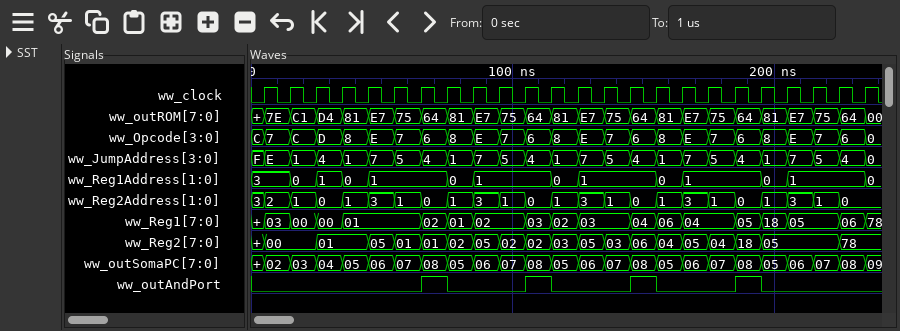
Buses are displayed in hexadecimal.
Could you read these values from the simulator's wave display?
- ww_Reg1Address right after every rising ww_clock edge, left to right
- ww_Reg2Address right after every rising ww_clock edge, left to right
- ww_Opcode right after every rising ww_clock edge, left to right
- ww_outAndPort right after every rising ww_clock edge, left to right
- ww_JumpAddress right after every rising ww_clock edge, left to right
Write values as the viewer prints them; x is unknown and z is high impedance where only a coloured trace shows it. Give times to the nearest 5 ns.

3, 0, 1, 0, 1, 1, 1, 0, 1, 1, 1, 0, 1, 1, 1, 0, 1, 1, 1, 0, 1, 1, 1, 0
2, 1, 0, 1, 3, 1, 0, 1, 3, 1, 0, 1, 3, 1, 0, 1, 3, 1, 0, 1, 3, 1, 0, 0
7, C, D, 8, E, 7, 6, 8, E, 7, 6, 8, E, 7, 6, 8, E, 7, 6, 8, E, 7, 6, 0
0 0 0 0 0 0 1 0 0 0 1 0 0 0 1 0 0 0 1 0 0 0 0 0
E, 1, 4, 1, 7, 5, 4, 1, 7, 5, 4, 1, 7, 5, 4, 1, 7, 5, 4, 1, 7, 5, 4, 0
